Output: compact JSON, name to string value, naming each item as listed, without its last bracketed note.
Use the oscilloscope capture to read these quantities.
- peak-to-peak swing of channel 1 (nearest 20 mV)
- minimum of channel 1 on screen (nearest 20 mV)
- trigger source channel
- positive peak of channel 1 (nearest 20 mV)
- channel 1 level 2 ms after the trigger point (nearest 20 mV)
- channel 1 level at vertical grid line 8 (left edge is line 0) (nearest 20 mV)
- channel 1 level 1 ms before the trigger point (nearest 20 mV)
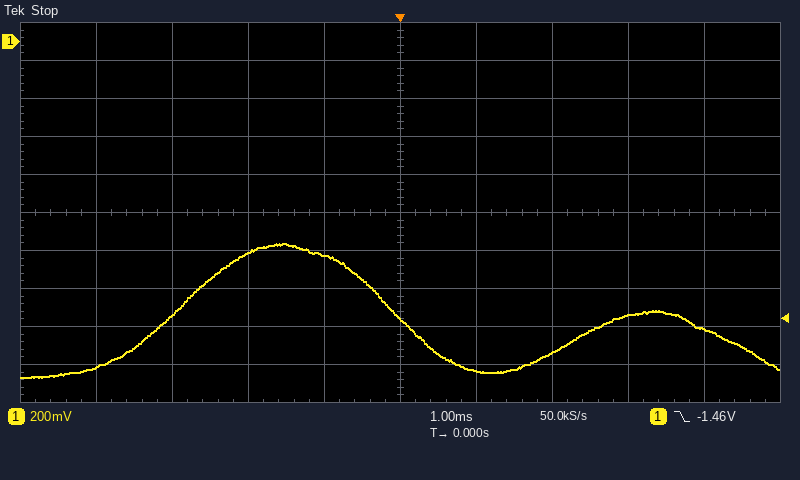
{"peak-to-peak swing of channel 1": "700 mV", "minimum of channel 1 on screen": "-1.76 V", "trigger source channel": "channel 1", "positive peak of channel 1": "-1.06 V", "channel 1 level 2 ms after the trigger point": "-1.64 V", "channel 1 level at vertical grid line 8 (left edge is line 0)": "-1.44 V", "channel 1 level 1 ms before the trigger point": "-1.12 V"}
